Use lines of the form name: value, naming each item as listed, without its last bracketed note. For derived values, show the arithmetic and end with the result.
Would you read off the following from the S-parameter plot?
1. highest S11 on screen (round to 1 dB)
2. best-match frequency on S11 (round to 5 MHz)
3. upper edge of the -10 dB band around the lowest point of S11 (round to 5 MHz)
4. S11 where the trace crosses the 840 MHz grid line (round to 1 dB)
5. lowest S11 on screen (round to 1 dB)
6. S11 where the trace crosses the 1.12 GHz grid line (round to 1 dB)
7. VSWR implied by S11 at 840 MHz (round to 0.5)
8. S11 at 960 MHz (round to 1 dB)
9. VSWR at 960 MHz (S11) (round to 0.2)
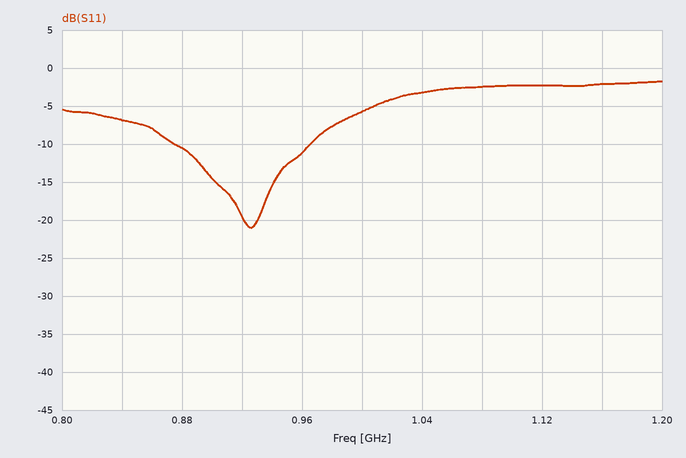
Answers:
highest S11 on screen: -2 dB
best-match frequency on S11: 925 MHz
upper edge of the -10 dB band around the lowest point of S11: 965 MHz
S11 where the trace crosses the 840 MHz grid line: -7 dB
lowest S11 on screen: -21 dB
S11 where the trace crosses the 1.12 GHz grid line: -2 dB
VSWR implied by S11 at 840 MHz: |Γ| = 10^(-7/20) = 0.4467; VSWR = (1 + 0.4467)/(1 − 0.4467) ≈ 2.61, so 2.5 to the nearest 0.5
S11 at 960 MHz: -11 dB
VSWR at 960 MHz (S11): |Γ| = 10^(-11/20) = 0.2818; VSWR = (1 + 0.2818)/(1 − 0.2818) ≈ 1.8
